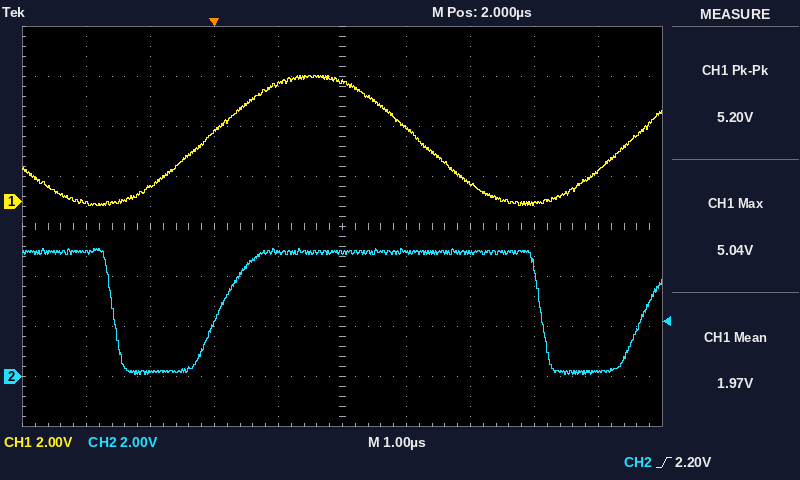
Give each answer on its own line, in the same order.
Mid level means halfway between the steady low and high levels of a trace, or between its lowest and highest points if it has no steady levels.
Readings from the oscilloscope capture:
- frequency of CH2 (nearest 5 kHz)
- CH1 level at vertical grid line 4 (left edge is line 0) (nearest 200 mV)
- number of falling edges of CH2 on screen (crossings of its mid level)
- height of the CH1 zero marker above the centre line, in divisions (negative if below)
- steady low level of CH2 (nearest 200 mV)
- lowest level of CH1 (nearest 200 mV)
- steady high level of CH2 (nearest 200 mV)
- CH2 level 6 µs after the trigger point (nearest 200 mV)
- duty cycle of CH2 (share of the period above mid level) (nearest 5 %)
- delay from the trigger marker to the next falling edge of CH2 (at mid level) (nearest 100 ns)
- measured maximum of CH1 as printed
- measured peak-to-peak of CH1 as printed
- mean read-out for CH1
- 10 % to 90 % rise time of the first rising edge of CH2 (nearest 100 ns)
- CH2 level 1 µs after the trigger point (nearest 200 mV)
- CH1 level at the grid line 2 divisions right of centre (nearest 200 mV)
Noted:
150 kHz
4.6 V
2
+0.5 div
200 mV
-200 mV
5.0 V
200 mV
75 %
5.1 µs
5.04 V
5.20 V
1.97 V
800 ns
5.0 V
800 mV
